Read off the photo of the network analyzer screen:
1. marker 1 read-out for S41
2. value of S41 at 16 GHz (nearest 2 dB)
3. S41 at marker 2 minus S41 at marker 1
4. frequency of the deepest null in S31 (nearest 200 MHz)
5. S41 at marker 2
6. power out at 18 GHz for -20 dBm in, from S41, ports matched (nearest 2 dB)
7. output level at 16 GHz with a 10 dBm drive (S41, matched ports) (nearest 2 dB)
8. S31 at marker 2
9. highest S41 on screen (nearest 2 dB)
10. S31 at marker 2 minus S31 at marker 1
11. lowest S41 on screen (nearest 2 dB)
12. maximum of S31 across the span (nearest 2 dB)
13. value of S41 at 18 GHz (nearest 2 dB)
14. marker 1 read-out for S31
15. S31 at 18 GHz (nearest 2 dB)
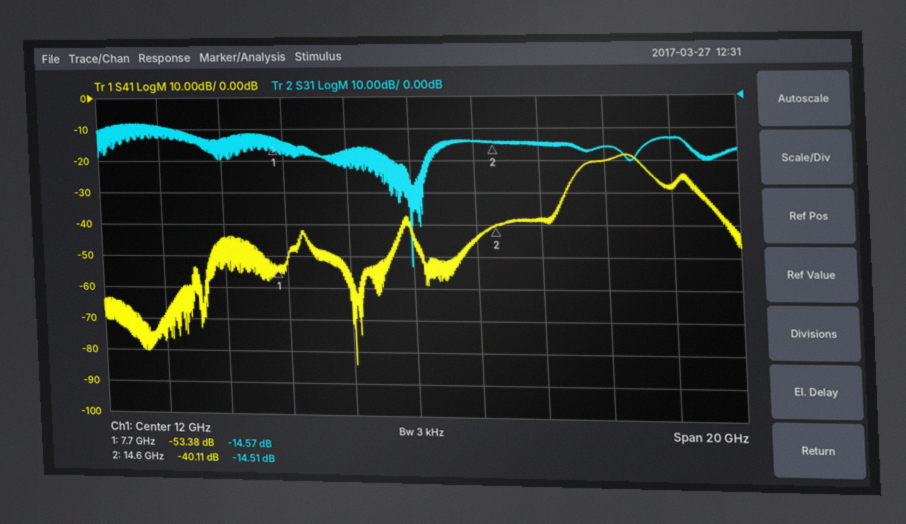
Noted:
-53.38 dB
-38 dB
13.27 dB
12.0 GHz
-40.11 dB
-40 dBm
-28 dBm
-14.51 dB
-18 dB
0.06 dB
-84 dB
-8 dB
-20 dB
-14.57 dB
-16 dB
